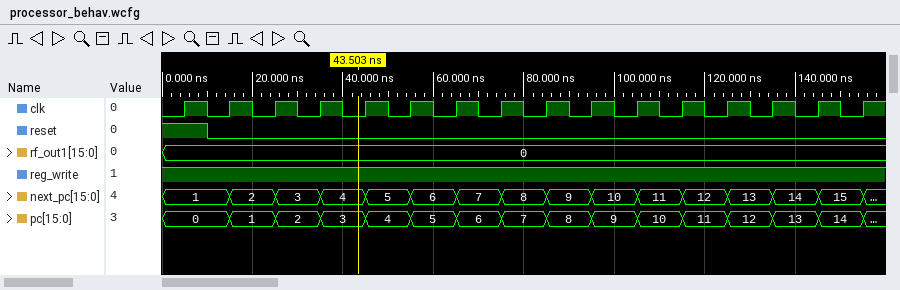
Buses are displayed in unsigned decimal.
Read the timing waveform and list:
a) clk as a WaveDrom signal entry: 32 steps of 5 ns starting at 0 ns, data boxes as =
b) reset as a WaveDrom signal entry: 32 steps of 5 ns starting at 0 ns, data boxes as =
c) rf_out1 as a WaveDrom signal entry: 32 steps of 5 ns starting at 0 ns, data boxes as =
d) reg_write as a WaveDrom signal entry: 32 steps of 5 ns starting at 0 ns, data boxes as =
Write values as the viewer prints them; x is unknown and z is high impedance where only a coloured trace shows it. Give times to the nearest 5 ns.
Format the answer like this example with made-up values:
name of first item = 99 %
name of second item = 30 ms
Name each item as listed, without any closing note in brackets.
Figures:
clk as a WaveDrom signal entry: 32 steps of 5 ns starting at 0 ns, data boxes as = = {name: 'clk', wave: '01010101010101010101010101010101'}
reset as a WaveDrom signal entry: 32 steps of 5 ns starting at 0 ns, data boxes as = = {name: 'reset', wave: '1.0.............................'}
rf_out1 as a WaveDrom signal entry: 32 steps of 5 ns starting at 0 ns, data boxes as = = {name: 'rf_out1', wave: '=...............................', data: '0'}
reg_write as a WaveDrom signal entry: 32 steps of 5 ns starting at 0 ns, data boxes as = = {name: 'reg_write', wave: '1...............................'}
